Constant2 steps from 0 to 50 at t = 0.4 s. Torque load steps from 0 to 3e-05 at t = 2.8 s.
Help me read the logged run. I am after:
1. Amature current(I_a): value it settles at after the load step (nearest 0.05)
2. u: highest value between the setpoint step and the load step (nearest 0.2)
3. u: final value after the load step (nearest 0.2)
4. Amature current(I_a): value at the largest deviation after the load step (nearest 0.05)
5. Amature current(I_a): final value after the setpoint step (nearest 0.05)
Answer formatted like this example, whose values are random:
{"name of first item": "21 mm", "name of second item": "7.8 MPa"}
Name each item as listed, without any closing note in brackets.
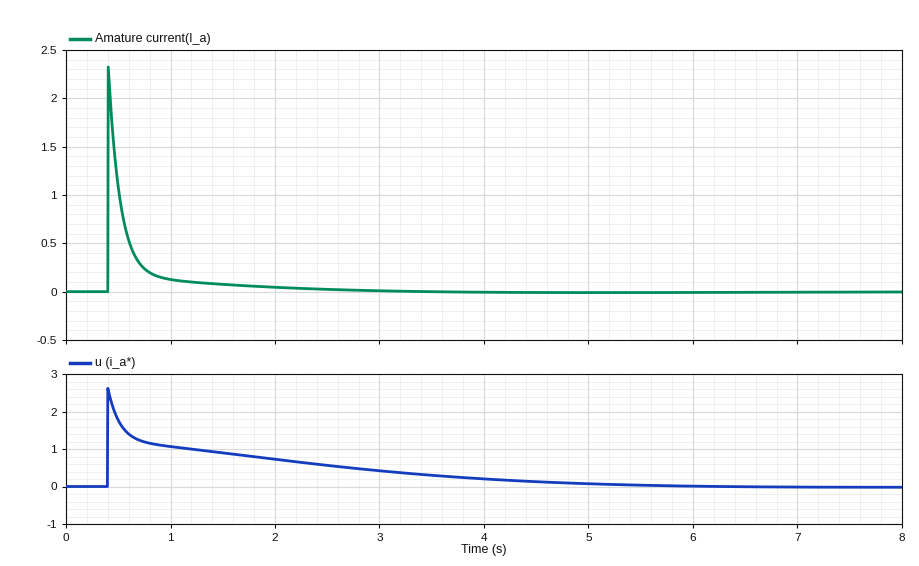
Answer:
{"Amature current(I_a): value it settles at after the load step": "0.00", "u: highest value between the setpoint step and the load step": "2.6", "u: final value after the load step": "0.0", "Amature current(I_a): value at the largest deviation after the load step": "0.00", "Amature current(I_a): final value after the setpoint step": "0.00"}
